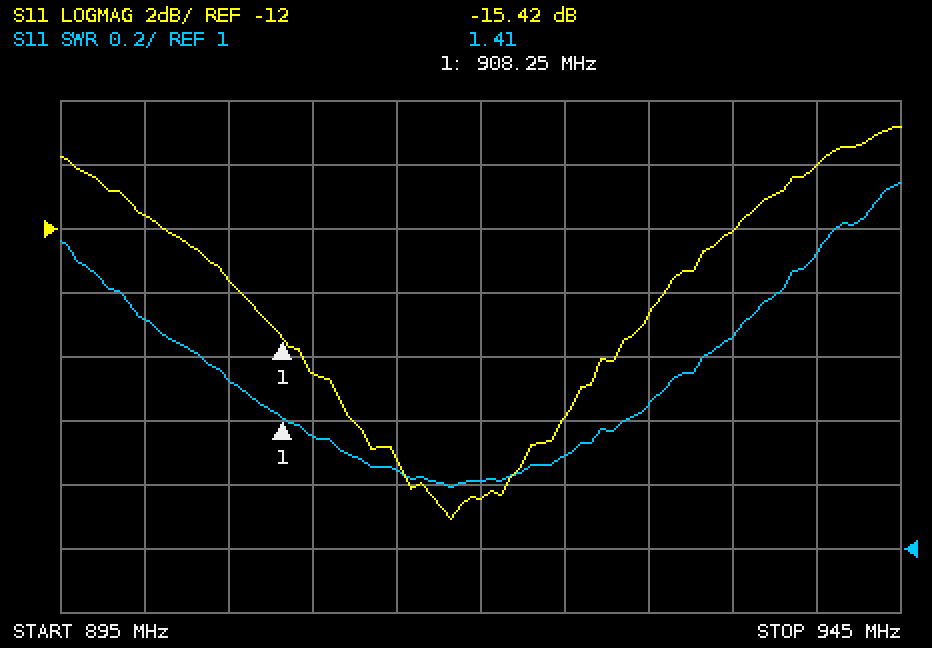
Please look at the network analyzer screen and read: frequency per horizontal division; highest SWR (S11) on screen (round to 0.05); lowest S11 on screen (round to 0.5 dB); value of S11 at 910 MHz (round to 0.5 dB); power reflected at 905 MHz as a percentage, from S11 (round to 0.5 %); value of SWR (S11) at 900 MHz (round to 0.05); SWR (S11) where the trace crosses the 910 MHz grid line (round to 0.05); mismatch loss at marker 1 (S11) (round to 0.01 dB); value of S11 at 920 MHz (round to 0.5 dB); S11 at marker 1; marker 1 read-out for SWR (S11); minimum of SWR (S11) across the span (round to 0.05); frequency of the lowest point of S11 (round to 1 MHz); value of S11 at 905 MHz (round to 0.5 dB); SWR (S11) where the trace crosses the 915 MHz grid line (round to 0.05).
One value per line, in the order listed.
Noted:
5 MHz
2.15
-21.0 dB
-16.5 dB
4.5 %
1.70
1.35
0.13 dB
-20.5 dB
-15.42 dB
1.41
1.20
918 MHz
-13.5 dB
1.25
